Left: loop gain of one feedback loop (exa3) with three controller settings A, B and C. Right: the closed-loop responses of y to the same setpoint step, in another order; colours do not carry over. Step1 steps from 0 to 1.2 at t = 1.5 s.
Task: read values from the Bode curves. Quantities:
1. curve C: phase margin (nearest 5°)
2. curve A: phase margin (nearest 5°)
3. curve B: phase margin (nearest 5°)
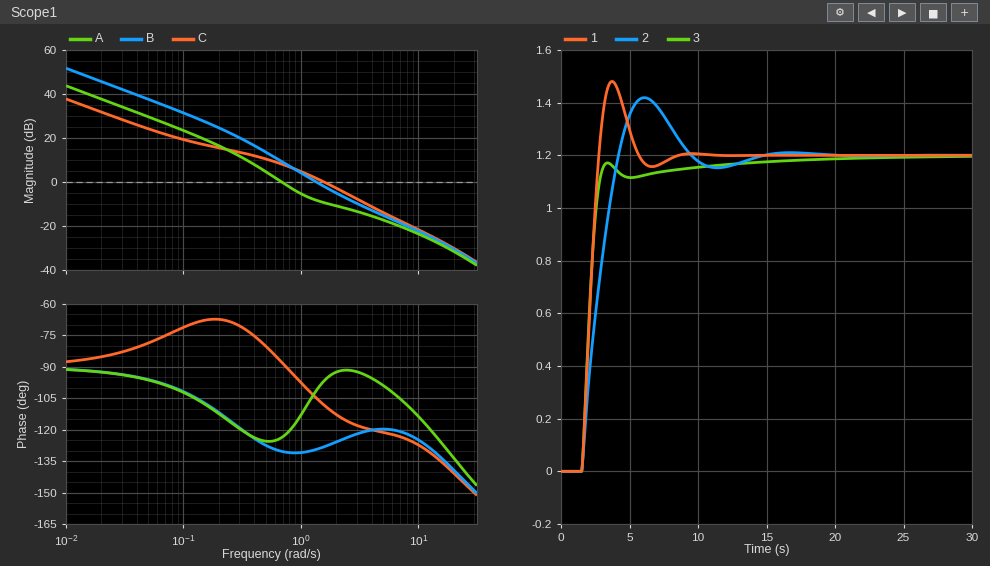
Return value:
70°
55°
50°
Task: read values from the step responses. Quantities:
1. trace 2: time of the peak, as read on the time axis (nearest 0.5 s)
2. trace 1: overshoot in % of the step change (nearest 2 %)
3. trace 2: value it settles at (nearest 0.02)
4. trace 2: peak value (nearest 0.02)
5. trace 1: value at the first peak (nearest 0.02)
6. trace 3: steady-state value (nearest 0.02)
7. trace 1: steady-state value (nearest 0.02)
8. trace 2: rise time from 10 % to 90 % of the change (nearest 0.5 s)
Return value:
6.0 s
24 %
1.20
1.42
1.48
1.20
1.20
2.0 s
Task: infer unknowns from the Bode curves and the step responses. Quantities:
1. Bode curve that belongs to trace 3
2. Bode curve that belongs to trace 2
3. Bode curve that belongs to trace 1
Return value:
C
A
B
